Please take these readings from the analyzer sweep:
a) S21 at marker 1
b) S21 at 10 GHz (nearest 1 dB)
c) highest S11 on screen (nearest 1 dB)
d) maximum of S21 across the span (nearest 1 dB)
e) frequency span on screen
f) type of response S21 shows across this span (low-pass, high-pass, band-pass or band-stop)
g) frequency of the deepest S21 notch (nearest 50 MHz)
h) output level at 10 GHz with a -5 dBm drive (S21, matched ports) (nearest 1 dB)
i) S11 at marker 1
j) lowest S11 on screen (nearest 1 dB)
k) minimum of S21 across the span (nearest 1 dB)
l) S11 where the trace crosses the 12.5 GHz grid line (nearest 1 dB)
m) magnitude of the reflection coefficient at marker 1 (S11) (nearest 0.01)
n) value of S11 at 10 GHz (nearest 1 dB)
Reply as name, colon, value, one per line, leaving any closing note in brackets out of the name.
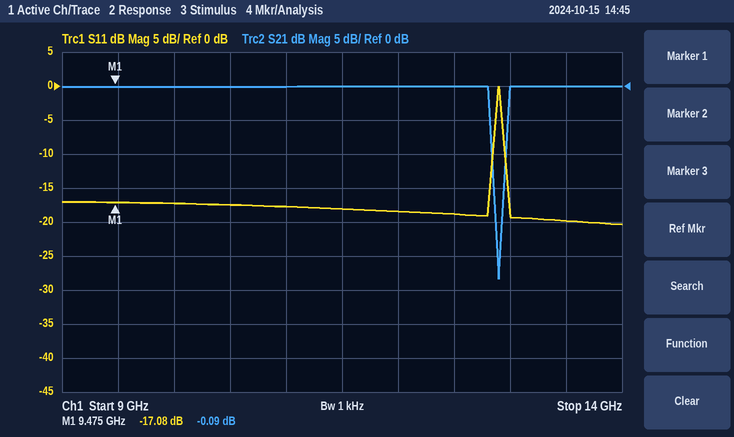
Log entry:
S21 at marker 1: -0.09 dB
S21 at 10 GHz: 0 dB
highest S11 on screen: 0 dB
maximum of S21 across the span: 0 dB
frequency span on screen: 5 GHz
type of response S21 shows across this span: band-stop
frequency of the deepest S21 notch: 12.90 GHz
output level at 10 GHz with a -5 dBm drive (S21, matched ports): -5 dBm
S11 at marker 1: -17.08 dB
lowest S11 on screen: -20 dB
minimum of S21 across the span: -28 dB
S11 where the trace crosses the 12.5 GHz grid line: -19 dB
magnitude of the reflection coefficient at marker 1 (S11): 0.14
value of S11 at 10 GHz: -17 dB
